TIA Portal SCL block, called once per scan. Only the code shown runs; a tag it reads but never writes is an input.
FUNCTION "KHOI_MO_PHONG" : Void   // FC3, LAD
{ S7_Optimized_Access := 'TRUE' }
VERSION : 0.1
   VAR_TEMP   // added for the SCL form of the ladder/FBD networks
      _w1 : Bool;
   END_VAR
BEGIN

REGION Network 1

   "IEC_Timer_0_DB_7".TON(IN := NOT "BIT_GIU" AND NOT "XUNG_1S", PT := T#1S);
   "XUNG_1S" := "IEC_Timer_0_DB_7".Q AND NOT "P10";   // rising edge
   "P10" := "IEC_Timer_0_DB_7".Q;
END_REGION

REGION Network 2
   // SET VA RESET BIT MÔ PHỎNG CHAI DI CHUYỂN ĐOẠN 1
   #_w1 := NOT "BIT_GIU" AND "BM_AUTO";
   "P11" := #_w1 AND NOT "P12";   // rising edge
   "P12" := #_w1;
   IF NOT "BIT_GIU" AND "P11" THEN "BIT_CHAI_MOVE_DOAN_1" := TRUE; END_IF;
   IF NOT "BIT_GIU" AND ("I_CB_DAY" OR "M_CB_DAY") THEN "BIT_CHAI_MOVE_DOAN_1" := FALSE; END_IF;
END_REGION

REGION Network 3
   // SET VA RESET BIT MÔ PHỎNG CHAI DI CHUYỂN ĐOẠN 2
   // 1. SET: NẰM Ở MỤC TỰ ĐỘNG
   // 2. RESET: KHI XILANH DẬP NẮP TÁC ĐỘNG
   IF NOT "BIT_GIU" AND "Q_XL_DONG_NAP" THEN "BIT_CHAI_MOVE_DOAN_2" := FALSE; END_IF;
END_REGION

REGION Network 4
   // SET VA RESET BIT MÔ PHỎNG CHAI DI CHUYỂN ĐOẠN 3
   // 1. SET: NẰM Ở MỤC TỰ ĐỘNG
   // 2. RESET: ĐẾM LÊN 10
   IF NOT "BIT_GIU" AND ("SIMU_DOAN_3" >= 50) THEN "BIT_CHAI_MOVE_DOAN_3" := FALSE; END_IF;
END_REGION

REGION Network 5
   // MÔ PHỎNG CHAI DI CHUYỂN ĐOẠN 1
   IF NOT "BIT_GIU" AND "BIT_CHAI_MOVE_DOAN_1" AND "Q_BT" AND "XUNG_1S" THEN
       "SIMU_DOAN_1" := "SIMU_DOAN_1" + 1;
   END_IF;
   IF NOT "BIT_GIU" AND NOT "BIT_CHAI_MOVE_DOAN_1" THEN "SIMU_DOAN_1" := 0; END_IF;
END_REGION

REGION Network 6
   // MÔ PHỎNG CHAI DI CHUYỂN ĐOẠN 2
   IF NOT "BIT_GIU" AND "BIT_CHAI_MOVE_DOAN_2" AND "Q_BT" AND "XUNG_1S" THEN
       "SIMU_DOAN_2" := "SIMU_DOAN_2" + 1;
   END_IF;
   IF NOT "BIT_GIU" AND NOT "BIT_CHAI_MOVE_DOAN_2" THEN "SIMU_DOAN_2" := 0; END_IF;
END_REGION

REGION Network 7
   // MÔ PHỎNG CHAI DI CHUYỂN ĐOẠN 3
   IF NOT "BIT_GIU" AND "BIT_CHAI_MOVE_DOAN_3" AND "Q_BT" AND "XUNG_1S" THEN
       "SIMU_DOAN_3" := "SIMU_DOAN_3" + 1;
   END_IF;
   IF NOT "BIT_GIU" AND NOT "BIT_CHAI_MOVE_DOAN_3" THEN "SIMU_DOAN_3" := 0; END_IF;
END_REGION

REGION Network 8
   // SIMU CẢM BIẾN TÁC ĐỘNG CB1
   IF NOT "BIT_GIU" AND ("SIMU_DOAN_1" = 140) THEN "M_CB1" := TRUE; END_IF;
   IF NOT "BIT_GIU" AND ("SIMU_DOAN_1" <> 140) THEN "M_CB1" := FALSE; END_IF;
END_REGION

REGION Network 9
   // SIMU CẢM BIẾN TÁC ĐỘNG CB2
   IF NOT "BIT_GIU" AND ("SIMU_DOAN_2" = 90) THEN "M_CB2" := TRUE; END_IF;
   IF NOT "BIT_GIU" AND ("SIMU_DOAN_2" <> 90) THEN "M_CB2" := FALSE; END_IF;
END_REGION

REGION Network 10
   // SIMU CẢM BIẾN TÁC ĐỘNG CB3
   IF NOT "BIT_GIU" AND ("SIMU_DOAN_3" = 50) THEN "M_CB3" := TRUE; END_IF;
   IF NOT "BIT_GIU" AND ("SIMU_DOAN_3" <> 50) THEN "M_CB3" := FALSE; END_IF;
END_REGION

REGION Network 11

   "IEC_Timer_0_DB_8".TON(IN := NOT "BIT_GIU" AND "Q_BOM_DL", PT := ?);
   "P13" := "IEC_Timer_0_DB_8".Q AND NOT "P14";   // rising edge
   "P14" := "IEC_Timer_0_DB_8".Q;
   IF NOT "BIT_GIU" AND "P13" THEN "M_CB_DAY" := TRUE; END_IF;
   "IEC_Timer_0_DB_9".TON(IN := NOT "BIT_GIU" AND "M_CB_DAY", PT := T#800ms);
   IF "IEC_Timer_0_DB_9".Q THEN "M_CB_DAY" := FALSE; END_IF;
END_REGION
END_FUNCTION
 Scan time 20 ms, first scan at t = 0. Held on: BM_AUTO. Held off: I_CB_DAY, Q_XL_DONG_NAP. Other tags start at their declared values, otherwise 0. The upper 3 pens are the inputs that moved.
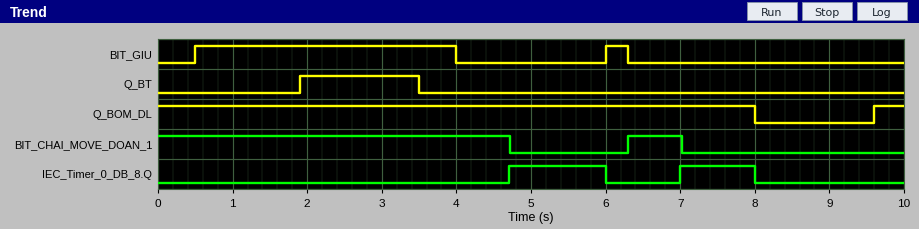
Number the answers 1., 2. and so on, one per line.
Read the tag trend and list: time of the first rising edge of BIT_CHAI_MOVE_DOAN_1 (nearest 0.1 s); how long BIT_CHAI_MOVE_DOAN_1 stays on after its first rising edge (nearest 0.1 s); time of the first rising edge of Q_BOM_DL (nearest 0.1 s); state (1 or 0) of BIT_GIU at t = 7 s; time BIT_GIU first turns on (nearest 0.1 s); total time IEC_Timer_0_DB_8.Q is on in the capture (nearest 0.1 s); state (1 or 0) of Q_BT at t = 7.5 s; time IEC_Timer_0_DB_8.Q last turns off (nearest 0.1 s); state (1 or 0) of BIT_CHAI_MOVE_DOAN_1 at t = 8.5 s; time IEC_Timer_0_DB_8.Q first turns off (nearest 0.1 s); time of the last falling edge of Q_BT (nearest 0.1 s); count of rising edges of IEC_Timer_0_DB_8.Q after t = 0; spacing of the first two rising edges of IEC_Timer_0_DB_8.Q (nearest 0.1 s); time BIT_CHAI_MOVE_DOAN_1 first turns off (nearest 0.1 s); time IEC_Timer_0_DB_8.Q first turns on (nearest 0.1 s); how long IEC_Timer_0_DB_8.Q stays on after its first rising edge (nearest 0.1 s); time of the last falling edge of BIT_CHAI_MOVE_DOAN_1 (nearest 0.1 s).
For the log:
1. 6.3 s
2. 0.7 s
3. 9.6 s
4. 0
5. 0.5 s
6. 2.3 s
7. 0
8. 8.0 s
9. 0
10. 6.0 s
11. 3.5 s
12. 2
13. 2.3 s
14. 4.7 s
15. 4.7 s
16. 1.3 s
17. 7.0 s
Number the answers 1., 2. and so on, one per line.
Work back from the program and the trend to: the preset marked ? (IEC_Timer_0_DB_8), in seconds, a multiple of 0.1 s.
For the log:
1. 0.7 s
